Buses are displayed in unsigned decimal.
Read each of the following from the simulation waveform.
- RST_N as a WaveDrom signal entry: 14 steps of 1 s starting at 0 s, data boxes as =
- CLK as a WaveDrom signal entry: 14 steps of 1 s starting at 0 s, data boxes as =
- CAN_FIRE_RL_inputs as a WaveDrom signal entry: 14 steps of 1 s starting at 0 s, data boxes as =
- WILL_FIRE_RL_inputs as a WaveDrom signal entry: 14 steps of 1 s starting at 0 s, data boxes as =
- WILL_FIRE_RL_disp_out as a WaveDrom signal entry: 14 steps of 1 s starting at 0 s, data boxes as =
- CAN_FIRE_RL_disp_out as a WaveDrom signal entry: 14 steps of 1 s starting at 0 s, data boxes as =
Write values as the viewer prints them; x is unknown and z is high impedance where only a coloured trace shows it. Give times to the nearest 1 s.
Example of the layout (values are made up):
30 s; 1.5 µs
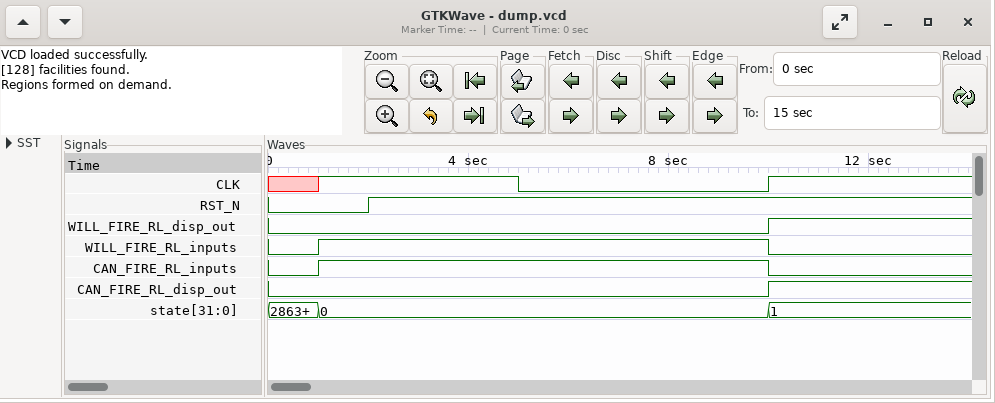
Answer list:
{name: 'RST_N', wave: '0.1...........'}; {name: 'CLK', wave: 'x1...0....1...'}; {name: 'CAN_FIRE_RL_inputs', wave: '01........0...'}; {name: 'WILL_FIRE_RL_inputs', wave: '01........0...'}; {name: 'WILL_FIRE_RL_disp_out', wave: '0.........1...'}; {name: 'CAN_FIRE_RL_disp_out', wave: '0.........1...'}
